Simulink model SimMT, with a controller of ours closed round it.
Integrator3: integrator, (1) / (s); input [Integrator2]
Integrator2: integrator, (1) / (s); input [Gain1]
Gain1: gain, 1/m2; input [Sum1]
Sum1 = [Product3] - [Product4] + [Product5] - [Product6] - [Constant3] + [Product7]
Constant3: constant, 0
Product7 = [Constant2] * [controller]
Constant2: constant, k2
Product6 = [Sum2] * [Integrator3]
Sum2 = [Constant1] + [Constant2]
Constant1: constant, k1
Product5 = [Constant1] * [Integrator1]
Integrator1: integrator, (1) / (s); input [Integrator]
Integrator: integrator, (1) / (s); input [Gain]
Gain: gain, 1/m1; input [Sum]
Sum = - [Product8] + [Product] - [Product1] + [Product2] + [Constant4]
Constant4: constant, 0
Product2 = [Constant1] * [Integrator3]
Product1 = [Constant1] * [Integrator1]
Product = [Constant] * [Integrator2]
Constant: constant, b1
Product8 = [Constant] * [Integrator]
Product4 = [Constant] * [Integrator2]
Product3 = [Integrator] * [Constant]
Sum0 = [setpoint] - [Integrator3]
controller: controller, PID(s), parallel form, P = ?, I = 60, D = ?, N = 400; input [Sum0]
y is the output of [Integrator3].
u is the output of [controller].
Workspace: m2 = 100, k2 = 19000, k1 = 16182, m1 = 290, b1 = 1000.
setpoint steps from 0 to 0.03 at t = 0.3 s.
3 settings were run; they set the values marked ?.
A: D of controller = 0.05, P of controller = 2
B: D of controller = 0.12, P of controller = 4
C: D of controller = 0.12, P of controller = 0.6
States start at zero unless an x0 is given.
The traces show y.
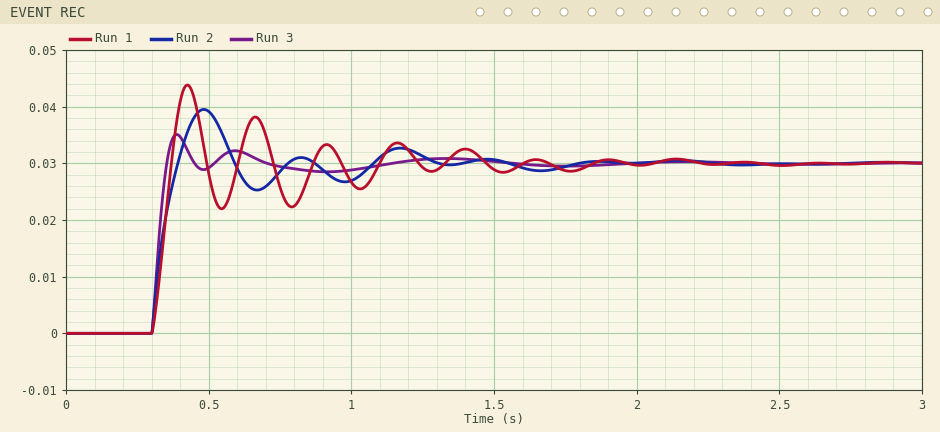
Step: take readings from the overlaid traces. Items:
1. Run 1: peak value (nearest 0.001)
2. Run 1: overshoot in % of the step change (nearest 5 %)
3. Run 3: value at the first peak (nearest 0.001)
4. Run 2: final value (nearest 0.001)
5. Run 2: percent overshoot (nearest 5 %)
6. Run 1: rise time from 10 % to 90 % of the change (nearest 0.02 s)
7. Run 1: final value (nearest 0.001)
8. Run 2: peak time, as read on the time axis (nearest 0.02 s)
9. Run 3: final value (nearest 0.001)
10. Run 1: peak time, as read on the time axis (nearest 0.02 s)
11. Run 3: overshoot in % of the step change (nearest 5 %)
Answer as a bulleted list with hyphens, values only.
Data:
- 0.044
- 45 %
- 0.035
- 0.030
- 30 %
- 0.06 s
- 0.030
- 0.48 s
- 0.030
- 0.42 s
- 15 %
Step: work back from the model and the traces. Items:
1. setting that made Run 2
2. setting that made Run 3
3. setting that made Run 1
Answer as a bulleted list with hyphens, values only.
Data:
- C
- B
- A
